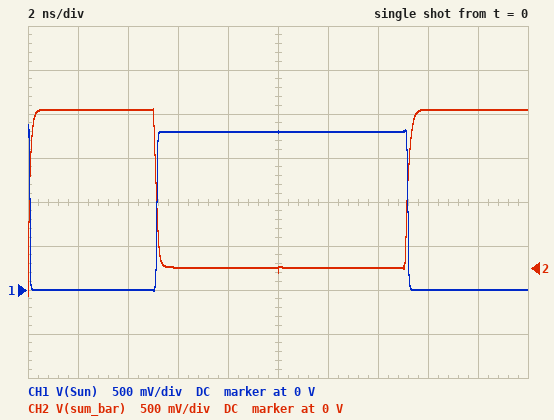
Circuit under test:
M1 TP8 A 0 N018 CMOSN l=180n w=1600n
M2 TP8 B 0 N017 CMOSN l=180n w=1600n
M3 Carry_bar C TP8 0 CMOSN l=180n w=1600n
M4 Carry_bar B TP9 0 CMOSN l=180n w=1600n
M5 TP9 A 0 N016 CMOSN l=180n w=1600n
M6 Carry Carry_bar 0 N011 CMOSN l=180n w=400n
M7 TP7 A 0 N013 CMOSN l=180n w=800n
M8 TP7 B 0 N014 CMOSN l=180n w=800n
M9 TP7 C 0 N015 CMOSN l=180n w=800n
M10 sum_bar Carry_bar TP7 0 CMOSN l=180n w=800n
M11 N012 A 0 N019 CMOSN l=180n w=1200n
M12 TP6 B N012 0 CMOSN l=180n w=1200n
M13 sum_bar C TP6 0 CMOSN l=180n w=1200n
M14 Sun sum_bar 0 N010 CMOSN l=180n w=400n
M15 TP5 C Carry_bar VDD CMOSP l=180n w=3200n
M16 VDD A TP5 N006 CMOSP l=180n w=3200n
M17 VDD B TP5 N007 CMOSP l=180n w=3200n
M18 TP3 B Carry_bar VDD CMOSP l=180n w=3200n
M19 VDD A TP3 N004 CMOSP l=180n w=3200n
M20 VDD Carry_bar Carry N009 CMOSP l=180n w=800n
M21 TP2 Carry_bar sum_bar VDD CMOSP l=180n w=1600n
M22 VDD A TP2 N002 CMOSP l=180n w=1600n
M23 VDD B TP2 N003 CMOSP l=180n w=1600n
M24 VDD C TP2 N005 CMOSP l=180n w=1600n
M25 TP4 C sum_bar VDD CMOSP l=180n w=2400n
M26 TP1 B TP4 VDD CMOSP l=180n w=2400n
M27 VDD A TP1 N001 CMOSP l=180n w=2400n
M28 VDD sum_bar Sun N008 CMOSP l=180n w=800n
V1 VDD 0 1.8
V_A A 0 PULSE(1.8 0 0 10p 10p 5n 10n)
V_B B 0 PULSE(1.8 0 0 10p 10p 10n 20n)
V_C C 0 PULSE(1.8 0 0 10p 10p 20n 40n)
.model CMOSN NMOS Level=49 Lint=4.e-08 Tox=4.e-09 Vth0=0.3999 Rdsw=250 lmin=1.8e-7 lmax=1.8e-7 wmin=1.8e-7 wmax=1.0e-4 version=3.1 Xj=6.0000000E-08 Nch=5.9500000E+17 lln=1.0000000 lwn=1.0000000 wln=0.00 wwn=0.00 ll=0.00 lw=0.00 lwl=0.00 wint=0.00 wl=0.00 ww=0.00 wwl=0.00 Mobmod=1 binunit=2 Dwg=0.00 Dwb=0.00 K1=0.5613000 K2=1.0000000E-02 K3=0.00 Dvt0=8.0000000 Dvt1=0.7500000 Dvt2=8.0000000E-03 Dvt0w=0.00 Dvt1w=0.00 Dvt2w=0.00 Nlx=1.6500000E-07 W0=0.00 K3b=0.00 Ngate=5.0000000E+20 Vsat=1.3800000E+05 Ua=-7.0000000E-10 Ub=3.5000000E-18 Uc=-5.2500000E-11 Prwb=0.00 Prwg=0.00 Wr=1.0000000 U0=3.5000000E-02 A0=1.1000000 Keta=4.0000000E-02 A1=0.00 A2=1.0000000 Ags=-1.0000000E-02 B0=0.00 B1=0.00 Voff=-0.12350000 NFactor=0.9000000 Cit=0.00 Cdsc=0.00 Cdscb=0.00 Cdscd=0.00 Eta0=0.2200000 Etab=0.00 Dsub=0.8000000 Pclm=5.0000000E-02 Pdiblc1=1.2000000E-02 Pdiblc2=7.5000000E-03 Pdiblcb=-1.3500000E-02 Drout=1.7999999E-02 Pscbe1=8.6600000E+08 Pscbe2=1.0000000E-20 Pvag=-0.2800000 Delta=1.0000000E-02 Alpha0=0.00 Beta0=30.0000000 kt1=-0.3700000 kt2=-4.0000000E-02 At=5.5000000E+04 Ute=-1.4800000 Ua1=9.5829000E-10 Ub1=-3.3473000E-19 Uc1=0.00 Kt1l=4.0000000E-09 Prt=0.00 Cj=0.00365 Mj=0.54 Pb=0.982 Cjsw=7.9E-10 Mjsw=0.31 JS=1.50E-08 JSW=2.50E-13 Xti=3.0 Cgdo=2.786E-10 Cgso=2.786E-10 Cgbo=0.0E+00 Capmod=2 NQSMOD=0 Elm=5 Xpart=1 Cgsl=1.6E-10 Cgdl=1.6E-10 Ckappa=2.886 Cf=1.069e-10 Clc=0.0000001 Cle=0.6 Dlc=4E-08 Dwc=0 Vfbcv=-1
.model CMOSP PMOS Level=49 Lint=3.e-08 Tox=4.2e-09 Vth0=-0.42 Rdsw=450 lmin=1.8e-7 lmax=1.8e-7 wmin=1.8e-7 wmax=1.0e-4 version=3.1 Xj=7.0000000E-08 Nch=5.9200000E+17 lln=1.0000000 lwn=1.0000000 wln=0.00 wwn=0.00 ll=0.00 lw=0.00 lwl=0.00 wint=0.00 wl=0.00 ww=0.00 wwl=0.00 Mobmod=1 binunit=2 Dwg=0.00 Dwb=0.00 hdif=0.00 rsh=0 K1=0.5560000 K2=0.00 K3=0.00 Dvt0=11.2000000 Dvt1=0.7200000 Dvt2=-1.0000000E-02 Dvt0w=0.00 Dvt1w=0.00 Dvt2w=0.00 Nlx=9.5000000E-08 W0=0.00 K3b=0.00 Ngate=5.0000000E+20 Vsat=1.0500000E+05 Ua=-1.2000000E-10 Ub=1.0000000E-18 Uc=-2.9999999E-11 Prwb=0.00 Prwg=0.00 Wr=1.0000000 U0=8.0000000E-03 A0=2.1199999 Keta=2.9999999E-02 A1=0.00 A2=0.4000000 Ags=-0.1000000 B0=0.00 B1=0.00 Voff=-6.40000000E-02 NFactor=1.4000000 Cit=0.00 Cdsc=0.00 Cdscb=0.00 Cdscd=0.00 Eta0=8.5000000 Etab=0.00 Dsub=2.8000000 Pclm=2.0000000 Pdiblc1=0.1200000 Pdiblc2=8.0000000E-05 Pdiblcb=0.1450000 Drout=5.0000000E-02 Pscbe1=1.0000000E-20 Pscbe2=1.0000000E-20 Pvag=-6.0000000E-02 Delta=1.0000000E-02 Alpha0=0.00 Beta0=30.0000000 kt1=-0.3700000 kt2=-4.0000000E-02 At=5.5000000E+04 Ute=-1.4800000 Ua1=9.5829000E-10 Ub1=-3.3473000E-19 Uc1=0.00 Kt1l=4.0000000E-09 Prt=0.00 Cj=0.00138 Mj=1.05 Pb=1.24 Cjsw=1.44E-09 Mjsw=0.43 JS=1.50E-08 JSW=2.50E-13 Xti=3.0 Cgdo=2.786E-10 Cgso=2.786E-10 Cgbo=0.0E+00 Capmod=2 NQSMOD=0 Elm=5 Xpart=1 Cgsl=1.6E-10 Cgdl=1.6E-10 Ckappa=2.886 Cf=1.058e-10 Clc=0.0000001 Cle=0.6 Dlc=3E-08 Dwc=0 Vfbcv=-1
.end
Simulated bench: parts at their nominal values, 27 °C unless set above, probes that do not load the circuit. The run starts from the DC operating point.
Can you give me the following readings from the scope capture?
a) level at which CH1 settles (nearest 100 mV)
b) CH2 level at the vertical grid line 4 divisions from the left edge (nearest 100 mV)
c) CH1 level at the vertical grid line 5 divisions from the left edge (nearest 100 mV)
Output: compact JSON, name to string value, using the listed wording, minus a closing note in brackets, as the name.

{"level at which CH1 settles": "0 V", "CH2 level at the vertical grid line 4 divisions from the left edge": "0 V", "CH1 level at the vertical grid line 5 divisions from the left edge": "1.8 V"}
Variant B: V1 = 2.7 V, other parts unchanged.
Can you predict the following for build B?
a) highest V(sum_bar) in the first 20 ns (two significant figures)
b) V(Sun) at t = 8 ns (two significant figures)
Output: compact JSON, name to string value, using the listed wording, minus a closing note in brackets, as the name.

{"highest V(sum_bar) in the first 20 ns": "2.7 V", "V(Sun) at t = 8 ns": "2.6 V"}
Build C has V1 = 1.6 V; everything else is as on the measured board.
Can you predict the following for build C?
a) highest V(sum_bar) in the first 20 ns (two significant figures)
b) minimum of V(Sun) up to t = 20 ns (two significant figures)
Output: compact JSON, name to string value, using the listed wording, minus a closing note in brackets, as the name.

{"highest V(sum_bar) in the first 20 ns": "1.6 V", "minimum of V(Sun) up to t = 20 ns": "-14 mV"}
